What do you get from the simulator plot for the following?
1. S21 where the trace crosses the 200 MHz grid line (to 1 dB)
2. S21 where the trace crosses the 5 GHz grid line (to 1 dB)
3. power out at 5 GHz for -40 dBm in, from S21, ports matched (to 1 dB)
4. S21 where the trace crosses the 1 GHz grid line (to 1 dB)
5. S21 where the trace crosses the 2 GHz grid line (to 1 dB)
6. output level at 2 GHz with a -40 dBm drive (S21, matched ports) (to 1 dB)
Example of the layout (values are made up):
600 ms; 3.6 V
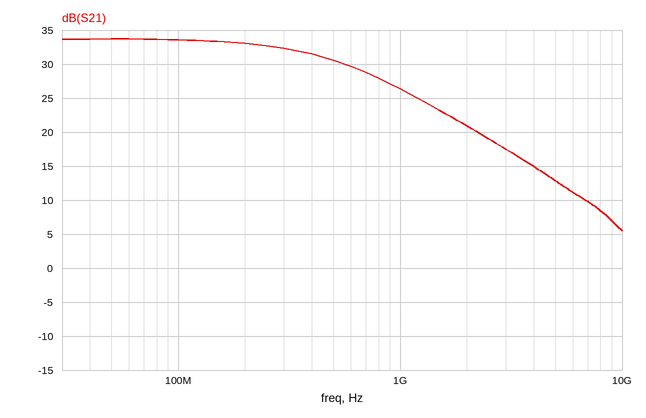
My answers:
33 dB; 13 dB; -27 dBm; 26 dB; 21 dB; -19 dBm
